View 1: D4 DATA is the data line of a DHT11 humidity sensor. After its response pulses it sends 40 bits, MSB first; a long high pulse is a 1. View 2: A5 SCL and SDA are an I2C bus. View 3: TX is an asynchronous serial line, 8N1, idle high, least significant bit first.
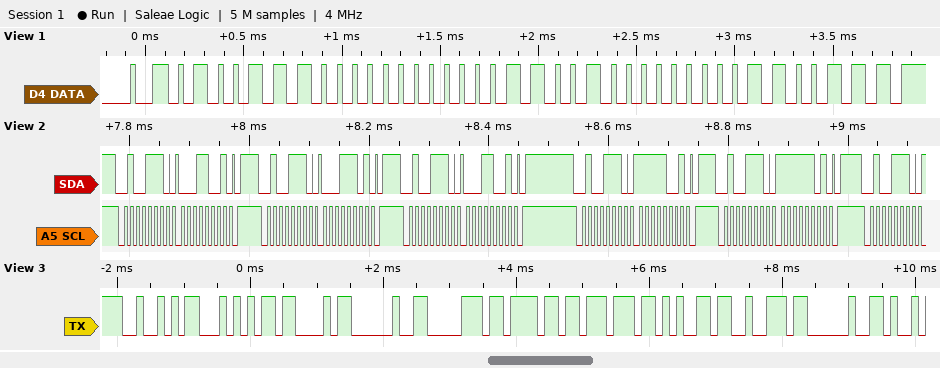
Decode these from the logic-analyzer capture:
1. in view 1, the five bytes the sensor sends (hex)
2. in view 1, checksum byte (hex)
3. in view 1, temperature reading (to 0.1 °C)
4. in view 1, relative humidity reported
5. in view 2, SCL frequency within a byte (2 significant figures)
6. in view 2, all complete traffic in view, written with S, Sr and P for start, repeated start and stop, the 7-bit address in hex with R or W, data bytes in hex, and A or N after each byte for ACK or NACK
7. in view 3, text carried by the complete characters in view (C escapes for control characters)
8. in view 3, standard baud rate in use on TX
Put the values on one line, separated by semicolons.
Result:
4E 00 19 00 67; 0x67; 25.0 °C; 78 %; 100 kHz; S 27W A 19 A P S 27W A 1D A P S 27W A 19 A P S 27W A F9 A P S 27W A FD A P S 27W A; "RTC power "; 9600 baud
